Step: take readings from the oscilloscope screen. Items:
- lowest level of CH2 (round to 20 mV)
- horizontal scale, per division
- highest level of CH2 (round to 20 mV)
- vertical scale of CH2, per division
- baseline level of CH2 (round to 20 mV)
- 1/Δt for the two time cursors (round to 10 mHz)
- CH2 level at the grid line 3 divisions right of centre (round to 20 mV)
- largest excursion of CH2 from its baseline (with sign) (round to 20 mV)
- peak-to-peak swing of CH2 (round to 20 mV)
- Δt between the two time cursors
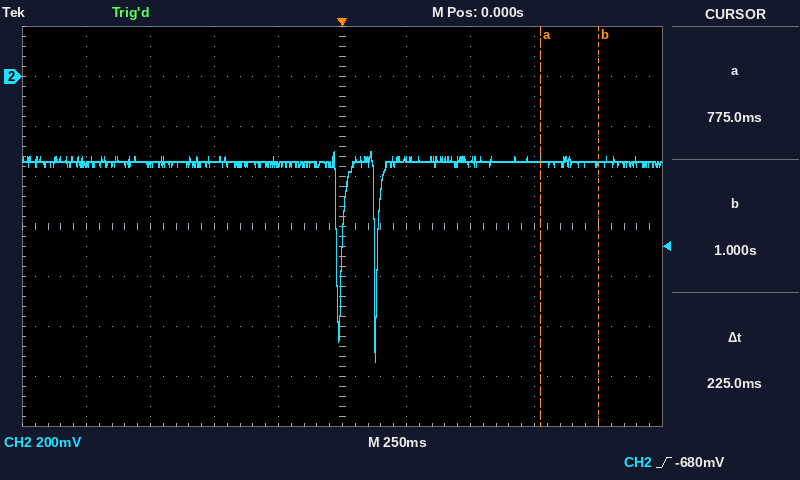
-1.14 V
250 ms
-300 mV
200 mV
-340 mV
4.44 Hz
-340 mV
-800 mV
840 mV
225 ms
